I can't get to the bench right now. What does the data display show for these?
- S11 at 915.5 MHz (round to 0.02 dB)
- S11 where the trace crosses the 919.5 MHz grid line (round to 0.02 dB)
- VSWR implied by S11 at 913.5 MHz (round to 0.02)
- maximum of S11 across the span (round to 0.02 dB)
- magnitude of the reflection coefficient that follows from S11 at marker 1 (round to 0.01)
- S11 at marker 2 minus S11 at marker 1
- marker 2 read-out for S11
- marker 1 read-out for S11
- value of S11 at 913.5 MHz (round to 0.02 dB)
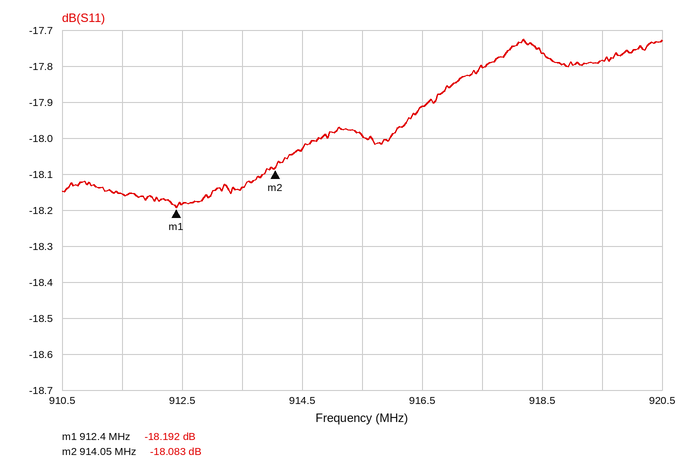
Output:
-18.00 dB
-17.78 dB
1.28
-17.72 dB
0.12
0.109 dB
-18.083 dB
-18.192 dB
-18.14 dB
